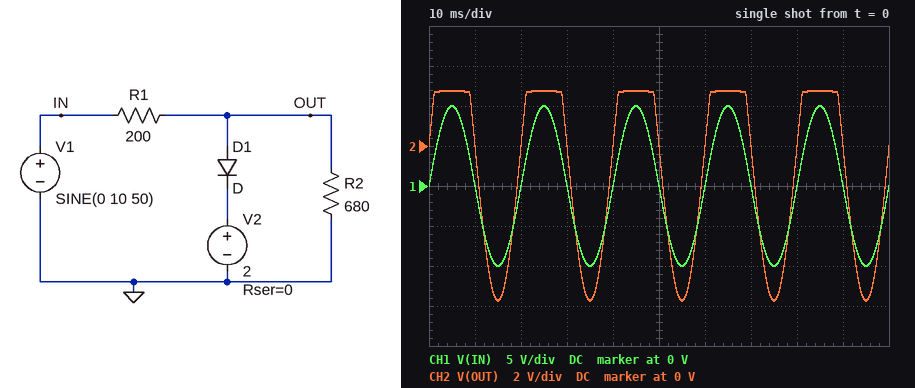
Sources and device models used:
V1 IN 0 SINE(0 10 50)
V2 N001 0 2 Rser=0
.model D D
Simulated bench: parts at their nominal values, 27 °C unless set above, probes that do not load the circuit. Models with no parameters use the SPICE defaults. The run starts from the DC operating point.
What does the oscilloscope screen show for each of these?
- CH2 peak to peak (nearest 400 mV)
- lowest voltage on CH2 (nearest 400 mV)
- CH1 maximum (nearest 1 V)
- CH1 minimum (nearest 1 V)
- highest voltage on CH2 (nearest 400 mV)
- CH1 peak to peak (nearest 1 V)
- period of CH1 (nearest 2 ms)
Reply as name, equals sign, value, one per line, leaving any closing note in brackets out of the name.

CH2 peak to peak = 10.4 V
lowest voltage on CH2 = -7.6 V
CH1 maximum = 10 V
CH1 minimum = -10 V
highest voltage on CH2 = 2.8 V
CH1 peak to peak = 20 V
period of CH1 = 20 ms
